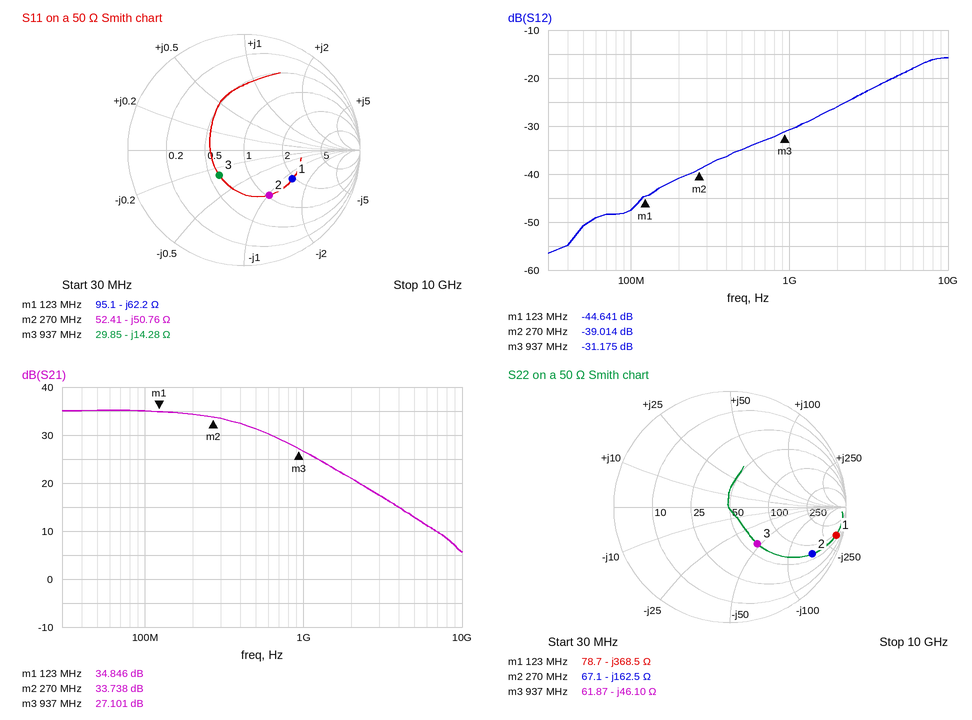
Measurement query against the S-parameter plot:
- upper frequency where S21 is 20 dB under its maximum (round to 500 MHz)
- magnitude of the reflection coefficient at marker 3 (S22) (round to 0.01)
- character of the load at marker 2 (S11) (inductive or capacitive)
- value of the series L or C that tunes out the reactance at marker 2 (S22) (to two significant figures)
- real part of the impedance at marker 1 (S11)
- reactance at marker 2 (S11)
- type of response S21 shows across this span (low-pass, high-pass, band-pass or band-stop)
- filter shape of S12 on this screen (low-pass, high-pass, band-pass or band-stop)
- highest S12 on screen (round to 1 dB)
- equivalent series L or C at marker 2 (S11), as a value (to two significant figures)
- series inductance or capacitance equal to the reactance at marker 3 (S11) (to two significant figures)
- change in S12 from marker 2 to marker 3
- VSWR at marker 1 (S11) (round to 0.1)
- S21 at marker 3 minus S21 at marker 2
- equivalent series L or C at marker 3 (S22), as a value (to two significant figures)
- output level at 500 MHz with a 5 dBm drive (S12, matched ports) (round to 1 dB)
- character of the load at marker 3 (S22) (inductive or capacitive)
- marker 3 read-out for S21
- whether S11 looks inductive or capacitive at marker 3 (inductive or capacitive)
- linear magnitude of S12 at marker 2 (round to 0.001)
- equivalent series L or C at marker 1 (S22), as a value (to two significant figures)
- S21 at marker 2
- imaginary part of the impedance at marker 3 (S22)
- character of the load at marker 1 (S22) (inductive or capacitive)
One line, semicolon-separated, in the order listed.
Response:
4.0 GHz; 0.39; capacitive; 96 nH; 95.1 Ω; -50.76 Ω; low-pass; high-pass; -16 dB; 12 pF; 12 pF; 7.839 dB; 2.9; -6.637 dB; 3.7 pF; -30 dBm; capacitive; 27.101 dB; capacitive; 0.011; 3.5 pF; 33.738 dB; -46.10 Ω; capacitive
